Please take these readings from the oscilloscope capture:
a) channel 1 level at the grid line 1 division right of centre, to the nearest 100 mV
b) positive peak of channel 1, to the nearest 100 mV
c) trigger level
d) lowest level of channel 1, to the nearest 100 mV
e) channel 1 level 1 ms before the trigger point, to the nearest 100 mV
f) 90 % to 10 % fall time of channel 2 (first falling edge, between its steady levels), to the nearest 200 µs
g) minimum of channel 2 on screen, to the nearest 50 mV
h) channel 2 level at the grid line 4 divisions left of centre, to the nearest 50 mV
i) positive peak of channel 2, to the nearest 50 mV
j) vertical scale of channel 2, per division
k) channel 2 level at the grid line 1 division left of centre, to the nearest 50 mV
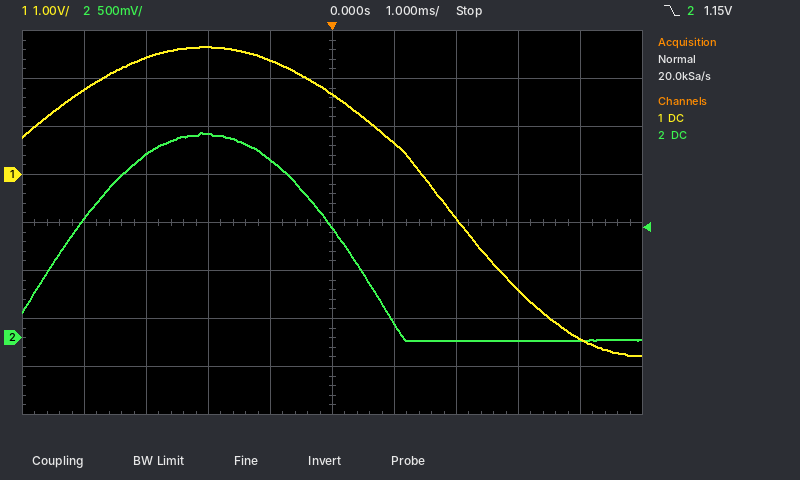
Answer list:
700 mV
2.7 V
1.15 V
-3.8 V
2.4 V
2.0 ms
-50 mV
1.25 V
2.15 V
500 mV
1.85 V
